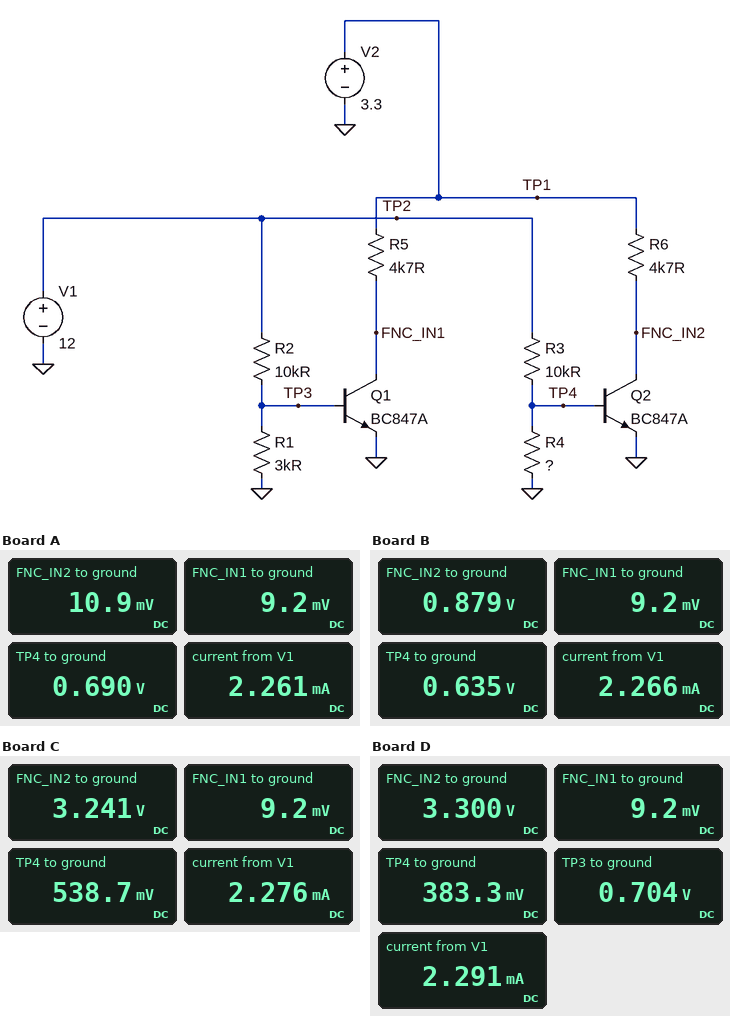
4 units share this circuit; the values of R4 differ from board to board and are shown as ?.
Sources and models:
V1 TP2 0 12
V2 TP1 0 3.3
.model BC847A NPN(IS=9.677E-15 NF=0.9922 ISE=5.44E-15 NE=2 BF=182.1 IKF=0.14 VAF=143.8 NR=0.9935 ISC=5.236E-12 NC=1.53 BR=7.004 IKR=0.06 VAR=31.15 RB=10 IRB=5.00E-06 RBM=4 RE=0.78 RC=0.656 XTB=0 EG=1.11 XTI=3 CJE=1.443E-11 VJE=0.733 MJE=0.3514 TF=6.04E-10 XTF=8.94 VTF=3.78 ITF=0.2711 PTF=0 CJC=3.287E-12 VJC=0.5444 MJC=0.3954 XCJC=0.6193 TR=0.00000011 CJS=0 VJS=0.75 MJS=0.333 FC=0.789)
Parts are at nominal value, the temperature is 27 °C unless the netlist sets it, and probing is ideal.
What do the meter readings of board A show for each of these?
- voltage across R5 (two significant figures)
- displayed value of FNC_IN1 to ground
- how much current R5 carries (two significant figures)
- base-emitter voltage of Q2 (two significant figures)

3.3 V
9.2 mV
700 µA
690 mV
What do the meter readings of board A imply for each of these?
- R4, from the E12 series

1.2 kΩ
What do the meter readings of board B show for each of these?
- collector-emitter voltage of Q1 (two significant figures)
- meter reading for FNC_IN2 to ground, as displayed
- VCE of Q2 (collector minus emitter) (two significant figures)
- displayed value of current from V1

9.2 mV
0.879 V
880 mV
2.266 mA
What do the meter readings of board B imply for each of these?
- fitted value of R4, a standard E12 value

560 Ω
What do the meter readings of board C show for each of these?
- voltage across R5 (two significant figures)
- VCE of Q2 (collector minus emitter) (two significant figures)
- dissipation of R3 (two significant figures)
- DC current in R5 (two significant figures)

3.3 V
3.2 V
13 mW
700 µA
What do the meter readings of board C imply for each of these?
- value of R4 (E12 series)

470 Ω
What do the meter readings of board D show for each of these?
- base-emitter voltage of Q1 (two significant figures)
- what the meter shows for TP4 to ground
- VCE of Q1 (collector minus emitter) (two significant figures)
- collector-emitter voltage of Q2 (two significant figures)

700 mV
383.3 mV
9.2 mV
3.3 V
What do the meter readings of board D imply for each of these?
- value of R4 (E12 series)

330 Ω
